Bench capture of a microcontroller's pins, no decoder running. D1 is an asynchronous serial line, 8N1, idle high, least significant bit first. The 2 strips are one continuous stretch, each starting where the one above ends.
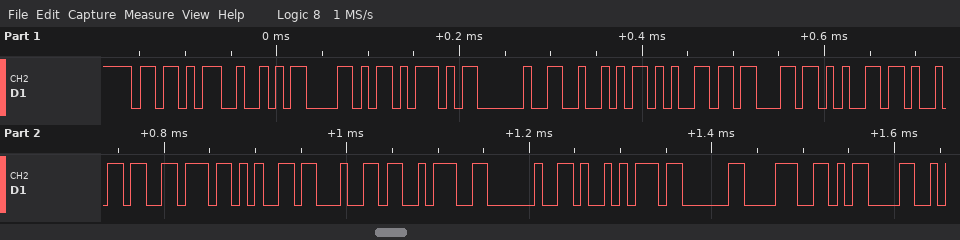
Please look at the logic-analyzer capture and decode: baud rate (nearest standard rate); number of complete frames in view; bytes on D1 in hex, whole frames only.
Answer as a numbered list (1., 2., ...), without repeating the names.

1. 115200 baud
2. 19
3. 5B 52 58 5D 20 52 65 63 65 69 76 65 64 3A 20 A9 03 38 0D
